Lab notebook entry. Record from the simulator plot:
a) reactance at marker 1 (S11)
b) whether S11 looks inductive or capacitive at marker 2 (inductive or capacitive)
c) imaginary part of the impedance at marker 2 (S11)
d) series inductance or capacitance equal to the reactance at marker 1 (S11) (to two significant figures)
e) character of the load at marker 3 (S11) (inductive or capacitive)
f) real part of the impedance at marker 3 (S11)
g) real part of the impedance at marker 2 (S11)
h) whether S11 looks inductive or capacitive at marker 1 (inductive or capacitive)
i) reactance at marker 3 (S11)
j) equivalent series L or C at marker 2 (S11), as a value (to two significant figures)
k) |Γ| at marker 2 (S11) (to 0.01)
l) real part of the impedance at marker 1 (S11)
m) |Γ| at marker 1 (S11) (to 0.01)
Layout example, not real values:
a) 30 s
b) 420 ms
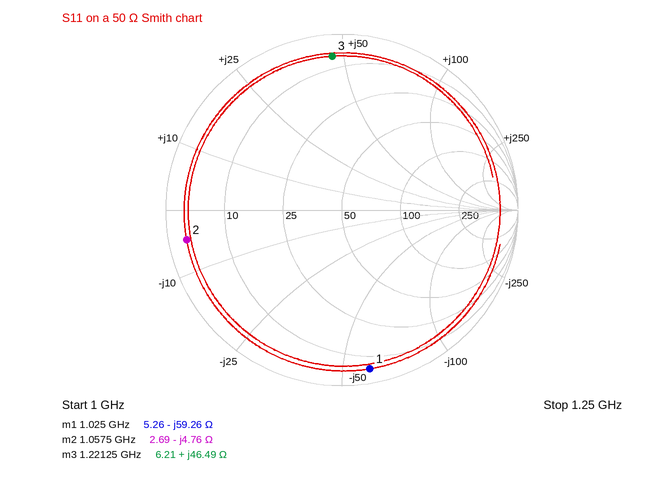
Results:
a) -59.26 Ω
b) capacitive
c) -4.76 Ω
d) 2.6 pF
e) inductive
f) 6.21 Ω
g) 2.69 Ω
h) capacitive
i) +46.49 Ω
j) 32 pF
k) 0.90
l) 5.26 Ω
m) 0.92
